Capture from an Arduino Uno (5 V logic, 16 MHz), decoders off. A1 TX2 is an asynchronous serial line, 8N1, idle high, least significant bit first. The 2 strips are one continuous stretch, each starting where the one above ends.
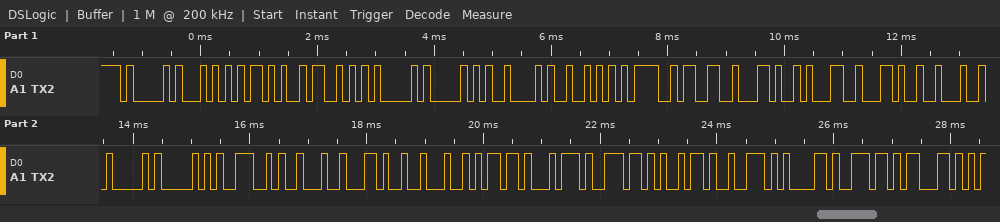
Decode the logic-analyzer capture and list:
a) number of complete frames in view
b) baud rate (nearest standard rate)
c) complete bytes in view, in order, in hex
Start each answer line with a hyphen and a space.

- 28
- 9600 baud
- 41 54 2B 53 41 50 42 52 3D 33 2C 31 2C 22 41 50 4E 22 2C 22 6D 74 6E 69 72 61 6E 63
